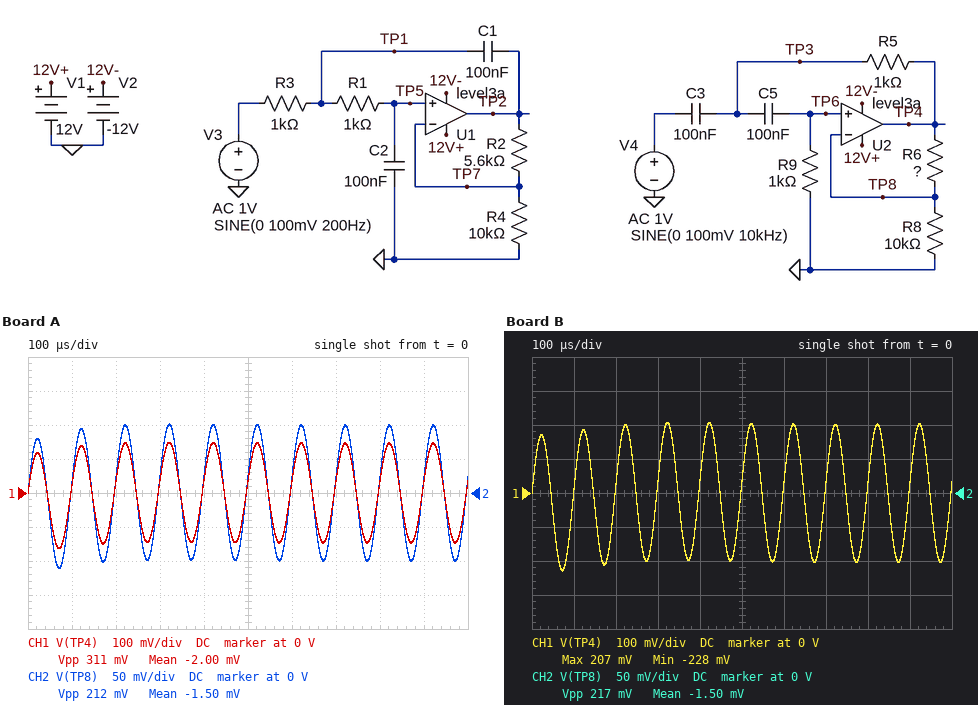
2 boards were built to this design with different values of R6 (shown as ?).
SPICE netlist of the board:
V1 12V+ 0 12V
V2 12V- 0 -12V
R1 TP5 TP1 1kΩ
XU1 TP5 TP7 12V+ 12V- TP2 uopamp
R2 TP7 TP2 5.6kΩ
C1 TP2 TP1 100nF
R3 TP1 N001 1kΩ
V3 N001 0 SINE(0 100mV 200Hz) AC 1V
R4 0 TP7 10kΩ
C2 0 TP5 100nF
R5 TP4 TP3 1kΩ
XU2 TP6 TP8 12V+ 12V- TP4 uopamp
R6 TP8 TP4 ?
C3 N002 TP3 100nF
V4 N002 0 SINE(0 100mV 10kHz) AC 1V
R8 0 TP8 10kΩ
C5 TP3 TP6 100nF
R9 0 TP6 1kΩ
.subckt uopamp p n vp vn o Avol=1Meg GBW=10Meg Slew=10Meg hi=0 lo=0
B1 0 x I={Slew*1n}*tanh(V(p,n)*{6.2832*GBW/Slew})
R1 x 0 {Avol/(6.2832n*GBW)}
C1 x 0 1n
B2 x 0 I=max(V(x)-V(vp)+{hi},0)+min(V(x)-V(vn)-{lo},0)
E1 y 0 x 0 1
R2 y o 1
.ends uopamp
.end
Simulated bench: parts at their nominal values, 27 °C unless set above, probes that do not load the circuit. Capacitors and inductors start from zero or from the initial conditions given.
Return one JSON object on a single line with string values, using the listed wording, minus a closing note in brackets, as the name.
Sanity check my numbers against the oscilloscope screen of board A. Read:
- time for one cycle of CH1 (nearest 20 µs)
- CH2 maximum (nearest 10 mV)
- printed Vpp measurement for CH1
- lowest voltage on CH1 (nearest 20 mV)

{"time for one cycle of CH1": "100 µs", "CH2 maximum": "100 mV", "printed Vpp measurement for CH1": "311 mV", "lowest voltage on CH1": "-160 mV"}
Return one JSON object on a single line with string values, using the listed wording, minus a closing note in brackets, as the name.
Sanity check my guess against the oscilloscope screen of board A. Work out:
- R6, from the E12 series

{"R6, from the E12 series": "4.7 kΩ"}
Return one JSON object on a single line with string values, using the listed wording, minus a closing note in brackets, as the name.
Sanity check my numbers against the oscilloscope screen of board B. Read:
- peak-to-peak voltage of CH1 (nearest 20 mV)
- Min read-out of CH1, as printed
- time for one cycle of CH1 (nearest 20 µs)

{"peak-to-peak voltage of CH1": "440 mV", "Min read-out of CH1, as printed": "-228 mV", "time for one cycle of CH1": "100 µs"}
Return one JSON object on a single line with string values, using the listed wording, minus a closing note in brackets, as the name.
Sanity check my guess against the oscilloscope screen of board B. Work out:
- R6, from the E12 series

{"R6, from the E12 series": "10 kΩ"}
